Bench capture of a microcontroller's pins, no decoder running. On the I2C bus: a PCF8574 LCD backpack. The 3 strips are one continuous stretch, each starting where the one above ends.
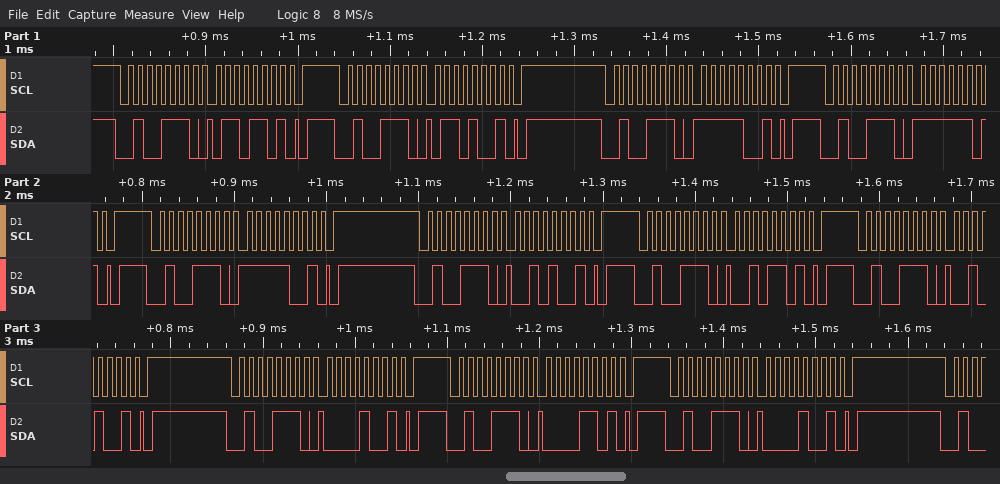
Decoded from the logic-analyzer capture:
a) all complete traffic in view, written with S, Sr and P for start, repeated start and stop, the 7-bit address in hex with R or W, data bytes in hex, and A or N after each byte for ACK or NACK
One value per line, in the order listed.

S 27W A 6D A P S 27W A 69 A P S 27W A F9 A P S 27W A FD A P S 27W A F9 A P S 27W A 29 A P S 27W A 2D A P S 27W A 29 A P S 27W A 09 A P S 27W A 0D A P S 27W A 09 A P
